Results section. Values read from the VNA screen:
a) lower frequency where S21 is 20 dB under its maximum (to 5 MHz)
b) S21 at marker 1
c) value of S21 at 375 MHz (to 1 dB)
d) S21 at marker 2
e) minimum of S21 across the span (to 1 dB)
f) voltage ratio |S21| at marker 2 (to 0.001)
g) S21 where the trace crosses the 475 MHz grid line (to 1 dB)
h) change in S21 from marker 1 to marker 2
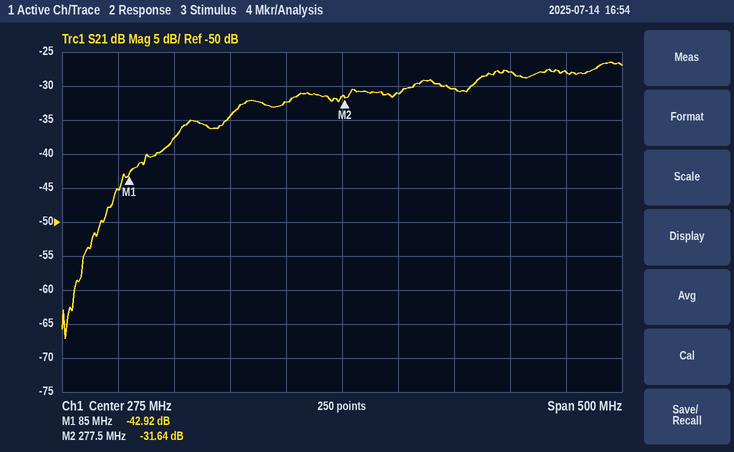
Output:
70 MHz
-42.92 dB
-30 dB
-31.64 dB
-67 dB
0.026
-28 dB
11.28 dB
